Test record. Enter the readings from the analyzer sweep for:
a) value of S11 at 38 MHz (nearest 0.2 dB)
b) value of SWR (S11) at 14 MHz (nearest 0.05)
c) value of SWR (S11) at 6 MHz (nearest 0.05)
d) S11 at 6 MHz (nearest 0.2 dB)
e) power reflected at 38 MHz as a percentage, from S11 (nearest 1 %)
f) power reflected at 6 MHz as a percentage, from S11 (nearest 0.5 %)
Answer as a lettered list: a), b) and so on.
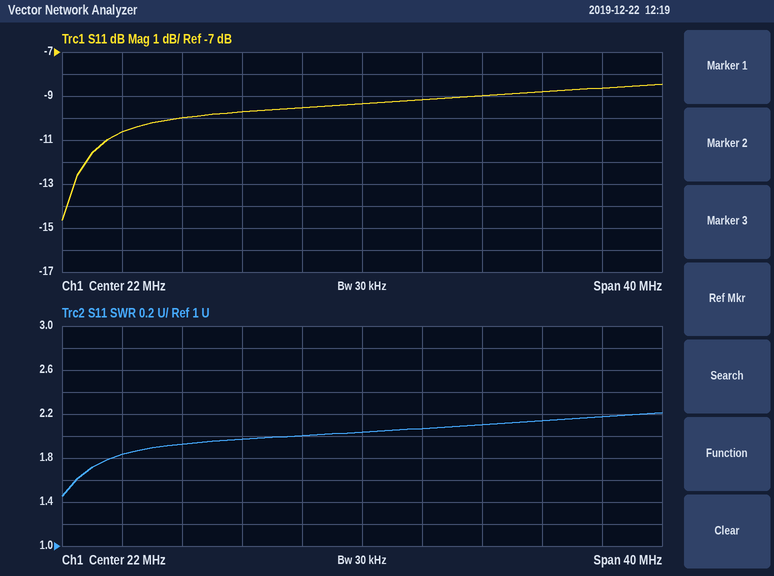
a) -8.6 dB
b) 1.95
c) 1.85
d) -10.6 dB
e) 14 %
f) 8.5 %
